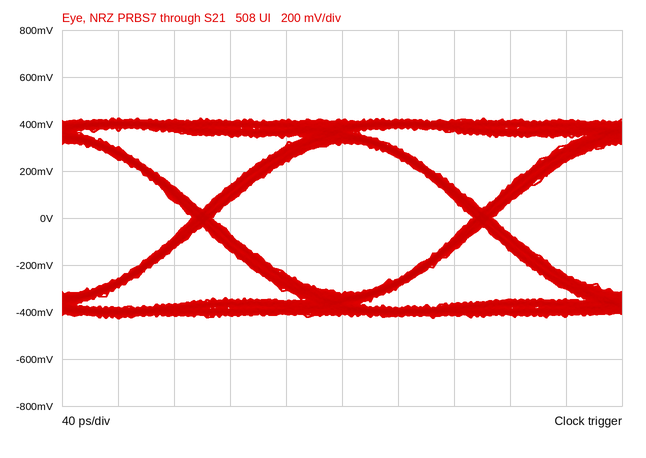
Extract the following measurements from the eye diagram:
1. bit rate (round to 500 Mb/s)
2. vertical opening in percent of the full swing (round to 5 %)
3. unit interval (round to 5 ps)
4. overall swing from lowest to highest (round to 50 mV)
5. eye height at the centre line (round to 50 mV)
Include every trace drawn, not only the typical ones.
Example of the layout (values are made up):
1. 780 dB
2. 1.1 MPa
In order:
1. 5.0 Gb/s
2. 75 %
3. 200 ps
4. 850 mV
5. 650 mV
